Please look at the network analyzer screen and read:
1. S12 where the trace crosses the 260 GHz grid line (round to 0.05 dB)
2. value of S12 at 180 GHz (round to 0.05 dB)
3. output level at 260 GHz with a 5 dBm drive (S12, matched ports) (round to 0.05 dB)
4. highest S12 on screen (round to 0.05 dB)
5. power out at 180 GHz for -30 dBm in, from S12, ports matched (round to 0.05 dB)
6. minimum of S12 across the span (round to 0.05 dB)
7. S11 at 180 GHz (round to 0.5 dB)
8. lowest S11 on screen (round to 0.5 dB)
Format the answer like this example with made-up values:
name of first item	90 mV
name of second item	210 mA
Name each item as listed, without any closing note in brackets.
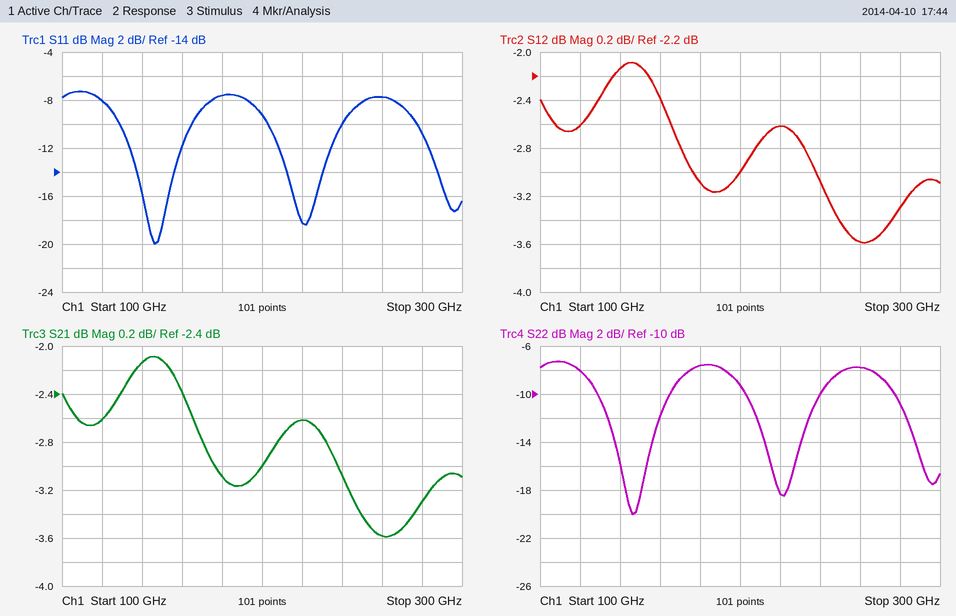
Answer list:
S12 where the trace crosses the 260 GHz grid line	-3.60 dB
value of S12 at 180 GHz	-3.10 dB
output level at 260 GHz with a 5 dBm drive (S12, matched ports)	1.40 dBm
highest S12 on screen	-2.10 dB
power out at 180 GHz for -30 dBm in, from S12, ports matched	-33.10 dBm
minimum of S12 across the span	-3.60 dB
S11 at 180 GHz	-7.5 dB
lowest S11 on screen	-20.0 dB
